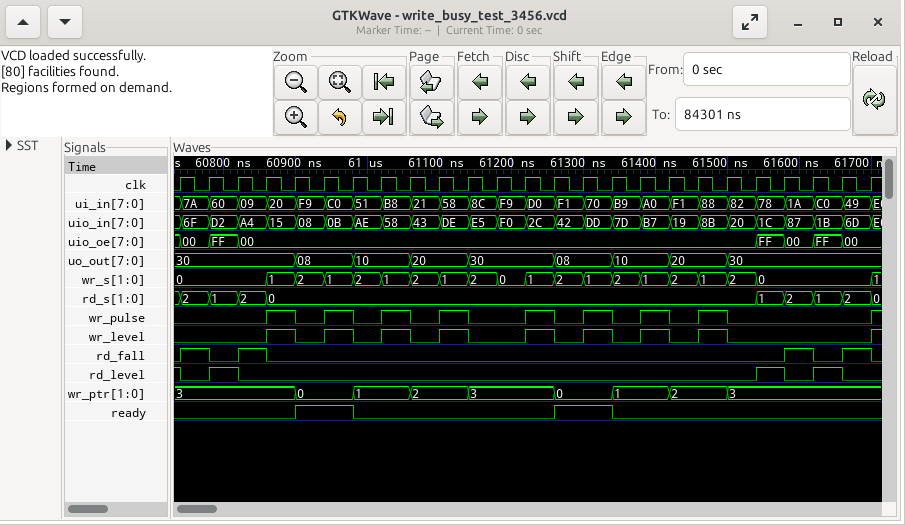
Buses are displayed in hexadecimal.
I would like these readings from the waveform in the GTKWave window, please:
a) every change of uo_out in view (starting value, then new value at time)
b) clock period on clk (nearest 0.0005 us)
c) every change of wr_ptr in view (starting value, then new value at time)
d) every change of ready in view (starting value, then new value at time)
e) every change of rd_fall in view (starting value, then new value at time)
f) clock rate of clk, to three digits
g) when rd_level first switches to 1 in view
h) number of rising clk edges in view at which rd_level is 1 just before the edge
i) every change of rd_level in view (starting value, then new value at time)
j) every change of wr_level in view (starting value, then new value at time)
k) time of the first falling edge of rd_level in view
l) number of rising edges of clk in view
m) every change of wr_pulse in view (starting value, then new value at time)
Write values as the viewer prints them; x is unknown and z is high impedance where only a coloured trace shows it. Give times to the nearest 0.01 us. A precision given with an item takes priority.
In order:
30, 08 at 60.9 us, 10 at 60.98 us, 20 at 61.06 us, 30 at 61.14 us, 08 at 61.26 us, 10 at 61.34 us, 20 at 61.42 us, 30 at 61.5 us
0.04 us
3, 0 at 60.9 us, 1 at 60.98 us, 2 at 61.06 us, 3 at 61.14 us, 0 at 61.26 us, 1 at 61.34 us, 2 at 61.42 us, 3 at 61.5 us
0, 1 at 60.9 us, 0 at 60.98 us, 1 at 61.26 us, 0 at 61.34 us
0, 1 at 60.74 us, 0 at 60.78 us, 1 at 60.82 us, 0 at 60.86 us, 1 at 61.58 us, 0 at 61.62 us, 1 at 61.66 us, 0 at 61.7 us
25.0 MHz
60.78 us
4
1, 0 at 60.74 us, 1 at 60.78 us, 0 at 60.82 us, 1 at 61.54 us, 0 at 61.58 us, 1 at 61.62 us, 0 at 61.66 us
0, 1 at 60.86 us, 0 at 60.9 us, 1 at 60.94 us, 0 at 60.98 us, 1 at 61.02 us, 0 at 61.06 us, 1 at 61.1 us, 0 at 61.14 us, 1 at 61.22 us, 0 at 61.26 us, 1 at 61.3 us, 0 at 61.34 us, 1 at 61.38 us, 0 at 61.42 us, 1 at 61.46 us, 0 at 61.5 us, 1 at 61.7 us
60.74 us
25
0, 1 at 60.86 us, 0 at 60.9 us, 1 at 60.94 us, 0 at 60.98 us, 1 at 61.02 us, 0 at 61.06 us, 1 at 61.1 us, 0 at 61.14 us, 1 at 61.22 us, 0 at 61.26 us, 1 at 61.3 us, 0 at 61.34 us, 1 at 61.38 us, 0 at 61.42 us, 1 at 61.46 us, 0 at 61.5 us, 1 at 61.7 us
